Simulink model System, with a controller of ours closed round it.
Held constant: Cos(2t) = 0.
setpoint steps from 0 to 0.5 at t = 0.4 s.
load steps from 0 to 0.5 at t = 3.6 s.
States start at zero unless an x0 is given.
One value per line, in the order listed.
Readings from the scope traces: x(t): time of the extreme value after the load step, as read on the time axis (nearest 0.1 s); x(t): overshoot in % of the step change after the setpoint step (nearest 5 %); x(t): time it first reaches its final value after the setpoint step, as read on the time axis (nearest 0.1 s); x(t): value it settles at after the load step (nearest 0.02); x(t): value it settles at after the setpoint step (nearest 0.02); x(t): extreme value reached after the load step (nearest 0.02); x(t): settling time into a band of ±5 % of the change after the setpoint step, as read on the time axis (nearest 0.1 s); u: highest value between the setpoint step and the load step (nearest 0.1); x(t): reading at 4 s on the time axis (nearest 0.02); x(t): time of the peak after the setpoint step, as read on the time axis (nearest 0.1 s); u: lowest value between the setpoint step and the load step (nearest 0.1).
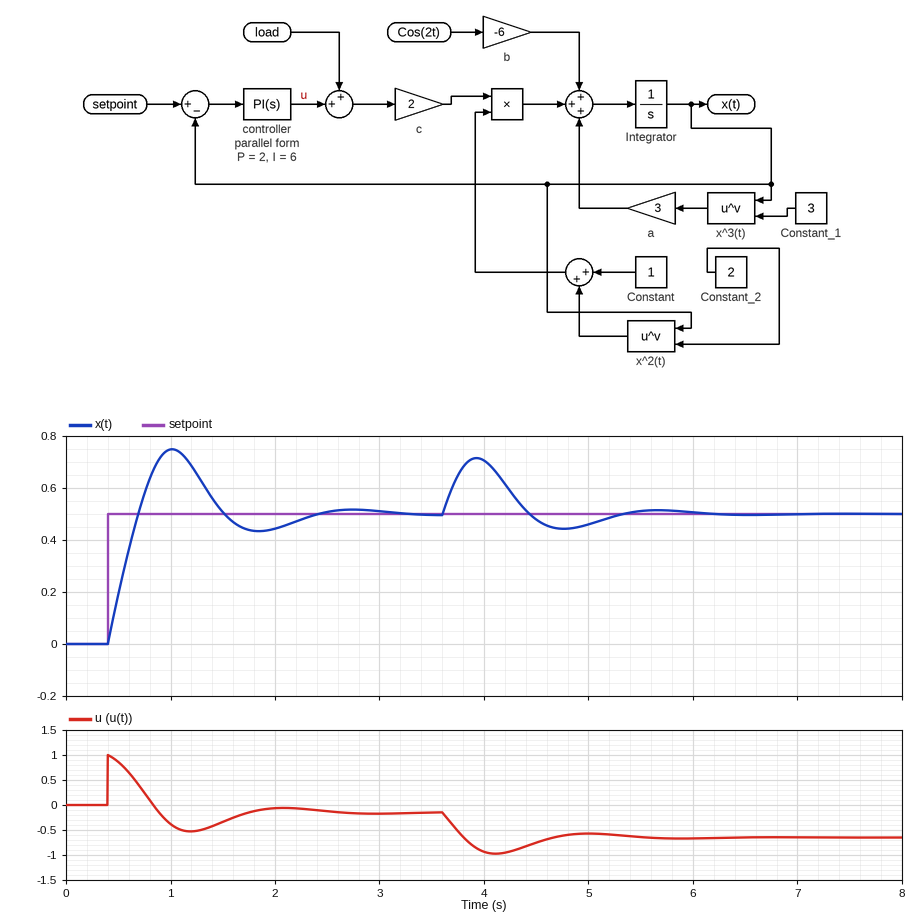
3.9 s
50 %
0.7 s
0.50
0.50
0.72
2.2 s
1.0
0.70
1.0 s
-0.5
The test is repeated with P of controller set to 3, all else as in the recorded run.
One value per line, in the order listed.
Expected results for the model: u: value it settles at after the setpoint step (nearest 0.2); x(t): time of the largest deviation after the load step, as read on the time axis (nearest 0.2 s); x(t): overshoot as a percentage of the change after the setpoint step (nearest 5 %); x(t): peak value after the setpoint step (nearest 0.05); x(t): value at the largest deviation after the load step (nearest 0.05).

-0.2
3.8 s
30 %
0.65
0.65
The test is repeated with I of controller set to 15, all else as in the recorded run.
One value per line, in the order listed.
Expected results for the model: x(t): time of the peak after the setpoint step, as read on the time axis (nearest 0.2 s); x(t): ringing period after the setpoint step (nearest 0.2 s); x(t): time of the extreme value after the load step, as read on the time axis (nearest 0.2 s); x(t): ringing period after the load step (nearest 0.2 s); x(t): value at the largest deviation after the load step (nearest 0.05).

0.8 s
1.0 s
3.8 s
1.0 s
0.65
